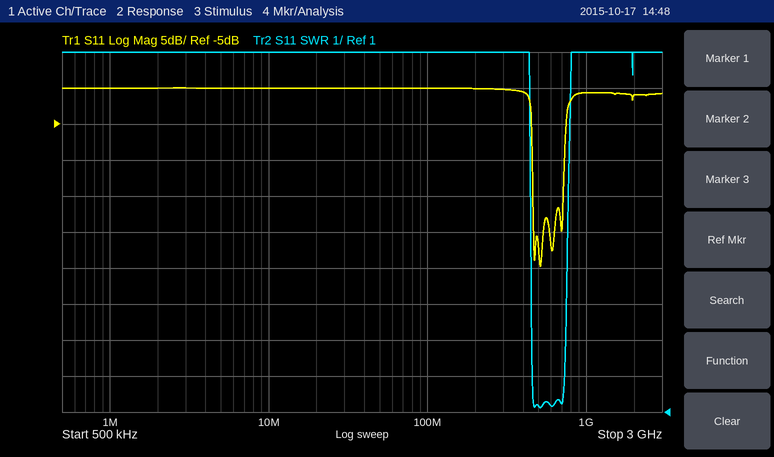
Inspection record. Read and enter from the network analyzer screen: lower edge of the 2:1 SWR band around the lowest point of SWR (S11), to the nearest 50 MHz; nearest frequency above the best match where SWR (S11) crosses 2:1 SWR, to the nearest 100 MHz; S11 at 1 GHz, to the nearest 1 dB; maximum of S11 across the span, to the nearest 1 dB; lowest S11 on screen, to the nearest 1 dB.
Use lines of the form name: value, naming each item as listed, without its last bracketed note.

lower edge of the 2:1 SWR band around the lowest point of SWR (S11), to the nearest 50 MHz: 450 MHz
nearest frequency above the best match where SWR (S11) crosses 2:1 SWR, to the nearest 100 MHz: 700 MHz
S11 at 1 GHz, to the nearest 1 dB: -1 dB
maximum of S11 across the span, to the nearest 1 dB: 0 dB
lowest S11 on screen, to the nearest 1 dB: -25 dB
